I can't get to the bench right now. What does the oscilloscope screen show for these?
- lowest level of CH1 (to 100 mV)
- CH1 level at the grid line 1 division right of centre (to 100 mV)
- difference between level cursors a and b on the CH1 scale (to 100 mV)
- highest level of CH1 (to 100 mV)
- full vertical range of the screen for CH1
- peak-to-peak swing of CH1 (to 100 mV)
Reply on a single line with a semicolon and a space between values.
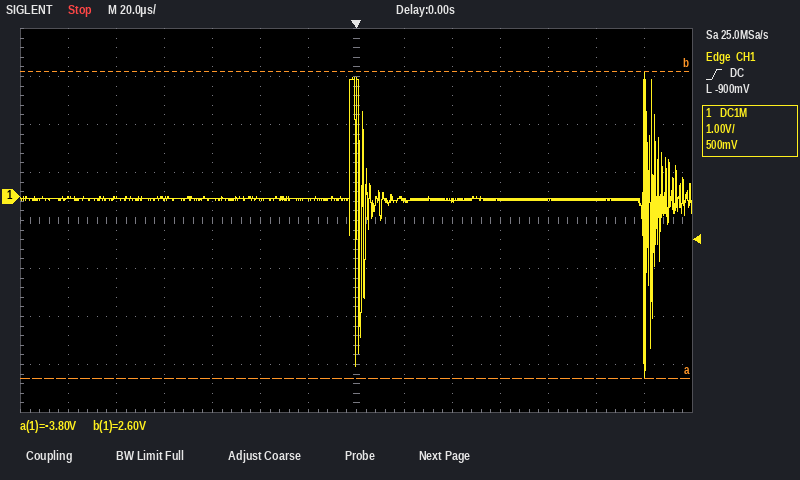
-3.8 V; -100 mV; 6.4 V; 2.6 V; 8 V; 6.4 V
